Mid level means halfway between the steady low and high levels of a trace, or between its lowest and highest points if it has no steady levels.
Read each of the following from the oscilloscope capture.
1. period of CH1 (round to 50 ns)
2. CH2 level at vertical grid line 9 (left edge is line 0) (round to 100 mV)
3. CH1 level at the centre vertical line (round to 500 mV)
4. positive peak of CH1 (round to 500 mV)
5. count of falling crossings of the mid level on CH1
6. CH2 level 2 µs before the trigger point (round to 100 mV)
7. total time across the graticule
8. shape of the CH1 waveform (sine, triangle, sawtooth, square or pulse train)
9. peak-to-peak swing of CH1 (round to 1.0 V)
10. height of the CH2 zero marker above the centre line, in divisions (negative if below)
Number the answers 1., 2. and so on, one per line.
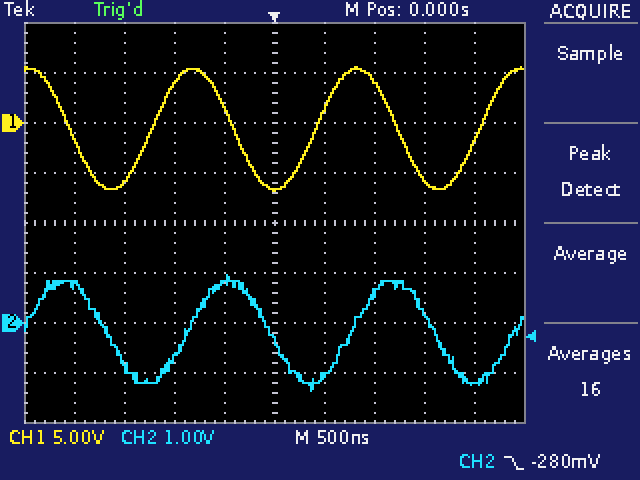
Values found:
1. 1.65 µs
2. -1.2 V
3. -6.5 V
4. 5.5 V
5. 3
6. 800 mV
7. 5 µs
8. sine
9. 12.0 V
10. -2.0 div
